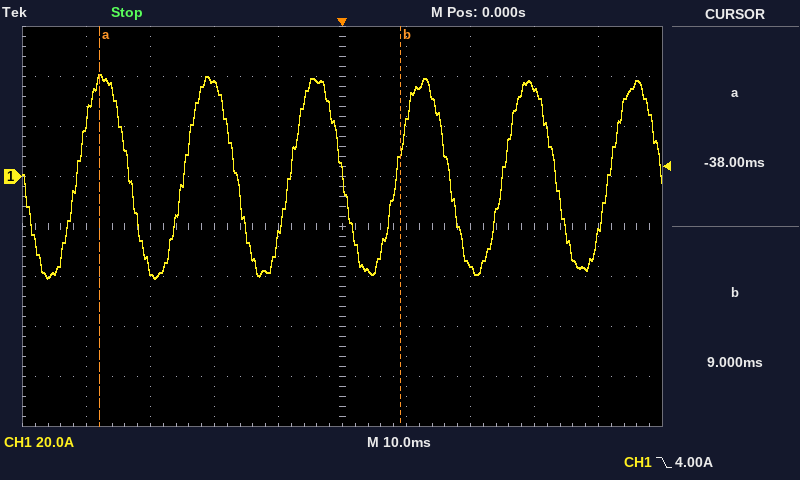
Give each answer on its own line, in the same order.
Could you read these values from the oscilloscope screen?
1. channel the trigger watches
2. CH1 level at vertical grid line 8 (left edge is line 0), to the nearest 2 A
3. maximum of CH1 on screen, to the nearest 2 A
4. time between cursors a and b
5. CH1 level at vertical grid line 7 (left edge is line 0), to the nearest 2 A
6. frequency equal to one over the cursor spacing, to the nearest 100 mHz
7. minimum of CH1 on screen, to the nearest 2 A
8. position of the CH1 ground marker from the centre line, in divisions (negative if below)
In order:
CH1
36 A
40 A
47 ms
-36 A
21.3 Hz
-40 A
+1.0 div
